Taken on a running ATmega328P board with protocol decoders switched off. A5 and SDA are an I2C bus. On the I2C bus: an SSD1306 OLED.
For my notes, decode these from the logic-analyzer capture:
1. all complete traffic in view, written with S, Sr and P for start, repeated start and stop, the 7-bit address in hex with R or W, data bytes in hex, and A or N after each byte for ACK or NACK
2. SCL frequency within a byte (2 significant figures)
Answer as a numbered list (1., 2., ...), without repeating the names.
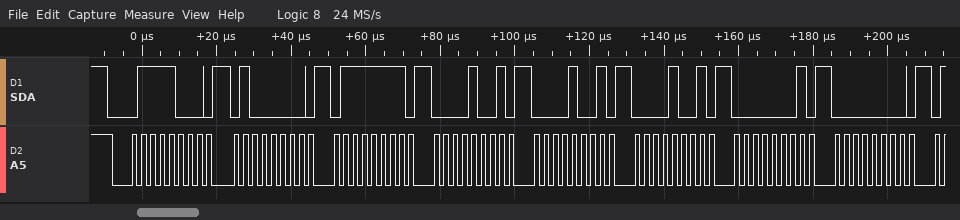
1. S 3CW A 40 A 7F A 09 A 09 A 09 A 01 A 00 A
2. 400 kHz
